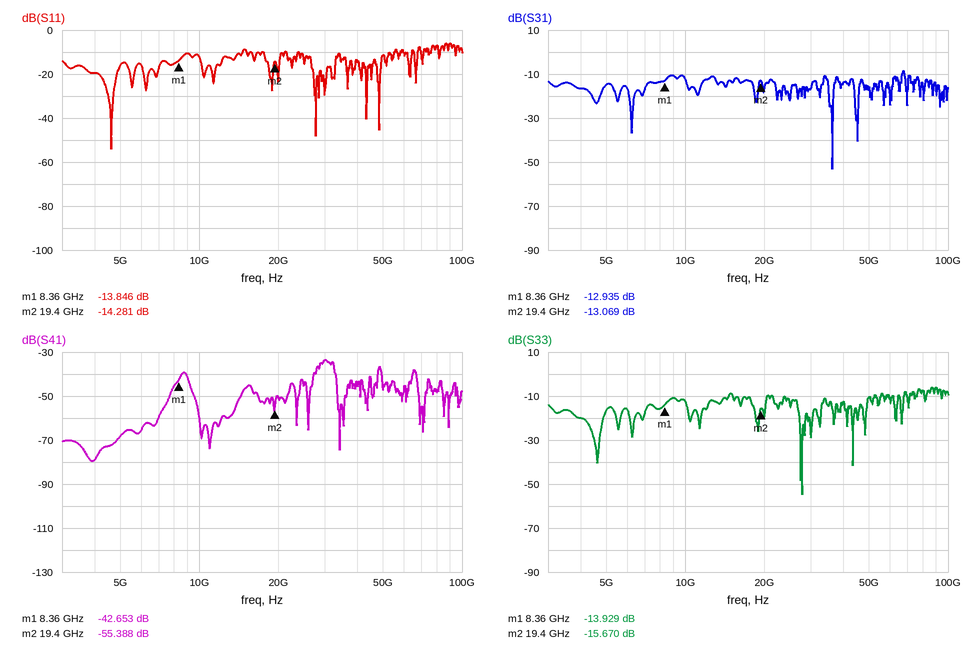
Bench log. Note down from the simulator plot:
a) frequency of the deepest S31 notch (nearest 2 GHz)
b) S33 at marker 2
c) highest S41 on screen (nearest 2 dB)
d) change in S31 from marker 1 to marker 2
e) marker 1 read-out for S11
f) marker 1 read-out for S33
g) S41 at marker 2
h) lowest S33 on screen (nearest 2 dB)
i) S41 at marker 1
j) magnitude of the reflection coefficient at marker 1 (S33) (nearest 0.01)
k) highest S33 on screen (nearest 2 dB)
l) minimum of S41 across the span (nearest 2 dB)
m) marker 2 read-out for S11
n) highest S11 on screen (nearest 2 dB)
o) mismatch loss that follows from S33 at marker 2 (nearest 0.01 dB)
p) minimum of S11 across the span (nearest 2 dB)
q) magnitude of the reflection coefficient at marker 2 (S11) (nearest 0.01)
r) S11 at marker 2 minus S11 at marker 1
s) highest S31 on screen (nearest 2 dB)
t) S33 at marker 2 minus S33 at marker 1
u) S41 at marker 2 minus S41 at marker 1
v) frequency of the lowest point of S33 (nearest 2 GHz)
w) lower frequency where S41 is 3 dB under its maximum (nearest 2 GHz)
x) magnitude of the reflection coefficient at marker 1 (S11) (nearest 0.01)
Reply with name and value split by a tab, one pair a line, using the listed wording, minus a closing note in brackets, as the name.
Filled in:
frequency of the deepest S31 notch	36 GHz
S33 at marker 2	-15.670 dB
highest S41 on screen	-34 dB
change in S31 from marker 1 to marker 2	-0.134 dB
marker 1 read-out for S11	-13.846 dB
marker 1 read-out for S33	-13.929 dB
S41 at marker 2	-55.388 dB
lowest S33 on screen	-54 dB
S41 at marker 1	-42.653 dB
magnitude of the reflection coefficient at marker 1 (S33)	0.20
highest S33 on screen	-6 dB
minimum of S41 across the span	-80 dB
marker 2 read-out for S11	-14.281 dB
highest S11 on screen	-6 dB
mismatch loss that follows from S33 at marker 2	0.12 dB
minimum of S11 across the span	-54 dB
magnitude of the reflection coefficient at marker 2 (S11)	0.19
S11 at marker 2 minus S11 at marker 1	-0.435 dB
highest S31 on screen	-8 dB
S33 at marker 2 minus S33 at marker 1	-1.741 dB
S41 at marker 2 minus S41 at marker 1	-12.735 dB
frequency of the lowest point of S33	28 GHz
lower frequency where S41 is 3 dB under its maximum	28 GHz
magnitude of the reflection coefficient at marker 1 (S11)	0.20
